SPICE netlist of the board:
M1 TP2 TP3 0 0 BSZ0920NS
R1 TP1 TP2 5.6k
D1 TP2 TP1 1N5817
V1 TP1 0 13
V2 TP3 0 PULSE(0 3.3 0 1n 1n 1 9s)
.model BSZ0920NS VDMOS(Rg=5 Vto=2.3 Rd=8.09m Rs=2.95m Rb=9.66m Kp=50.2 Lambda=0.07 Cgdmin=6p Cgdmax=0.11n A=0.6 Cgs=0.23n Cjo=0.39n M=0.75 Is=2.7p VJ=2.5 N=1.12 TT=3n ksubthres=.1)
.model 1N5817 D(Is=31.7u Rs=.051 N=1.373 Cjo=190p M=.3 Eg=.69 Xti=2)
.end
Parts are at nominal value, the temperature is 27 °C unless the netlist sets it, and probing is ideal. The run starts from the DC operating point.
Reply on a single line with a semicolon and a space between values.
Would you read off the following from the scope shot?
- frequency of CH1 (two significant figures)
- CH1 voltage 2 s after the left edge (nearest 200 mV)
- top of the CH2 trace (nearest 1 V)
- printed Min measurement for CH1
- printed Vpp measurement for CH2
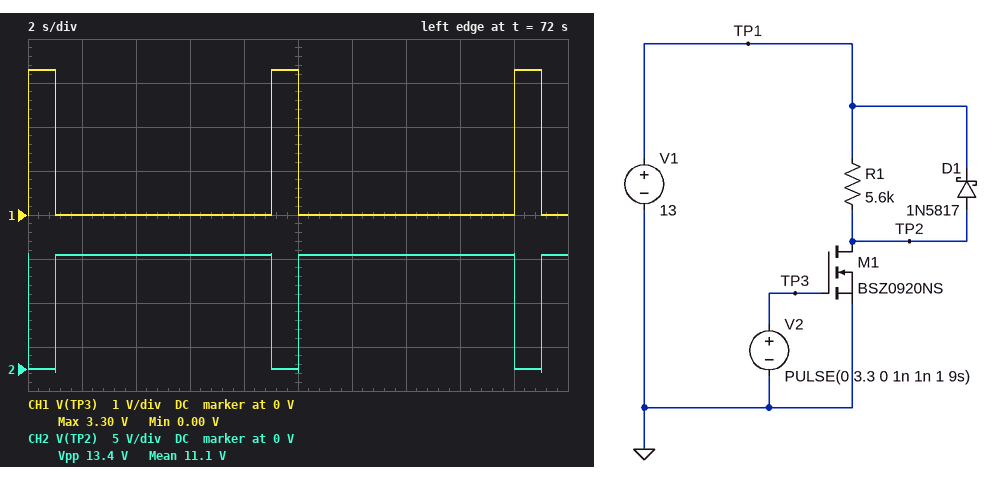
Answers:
110 mHz; 0 V; 13 V; 0.00 V; 13.4 V
